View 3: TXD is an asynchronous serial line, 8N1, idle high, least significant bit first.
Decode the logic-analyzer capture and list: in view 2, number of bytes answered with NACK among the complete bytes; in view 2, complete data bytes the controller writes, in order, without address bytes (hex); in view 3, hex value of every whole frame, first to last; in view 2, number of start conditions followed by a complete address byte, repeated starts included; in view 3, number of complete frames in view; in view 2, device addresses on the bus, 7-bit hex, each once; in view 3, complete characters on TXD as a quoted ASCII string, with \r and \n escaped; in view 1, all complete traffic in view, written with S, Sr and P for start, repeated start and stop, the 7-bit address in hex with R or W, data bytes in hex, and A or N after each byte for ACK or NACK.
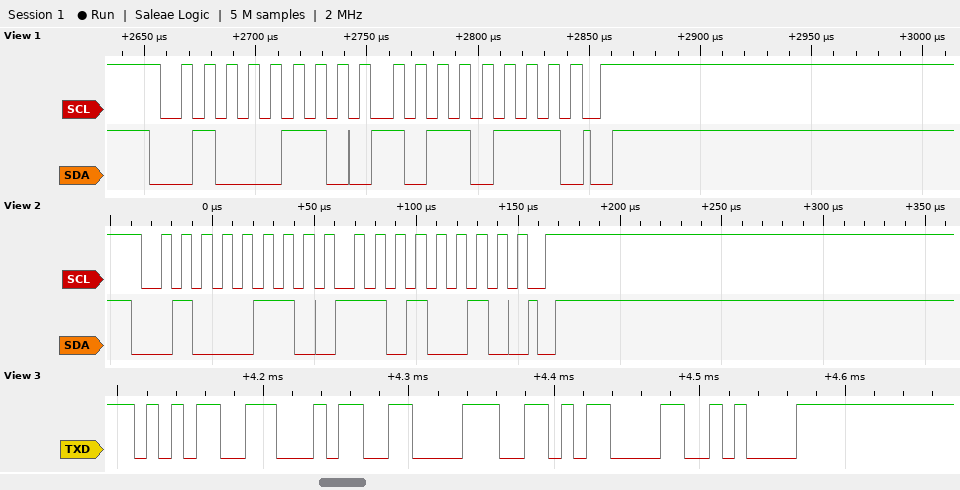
0
D2
35 34 38 0D 0A
1
5
0x23
"548\r\n"
S 23W A B7 A P
